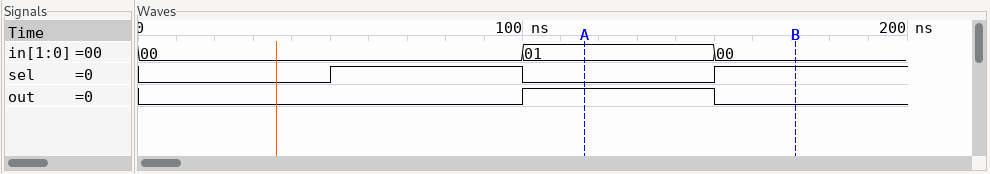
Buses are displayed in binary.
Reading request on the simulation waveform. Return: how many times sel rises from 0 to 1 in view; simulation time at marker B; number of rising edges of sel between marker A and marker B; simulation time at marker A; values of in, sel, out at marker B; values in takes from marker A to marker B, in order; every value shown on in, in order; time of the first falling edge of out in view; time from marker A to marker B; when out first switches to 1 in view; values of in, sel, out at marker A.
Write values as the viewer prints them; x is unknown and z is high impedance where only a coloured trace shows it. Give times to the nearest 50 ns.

2
150 ns
1
100 ns
in=00, sel=1, out=0
01, 00
00, 01, 00
150 ns
50 ns
100 ns
in=01, sel=0, out=1
